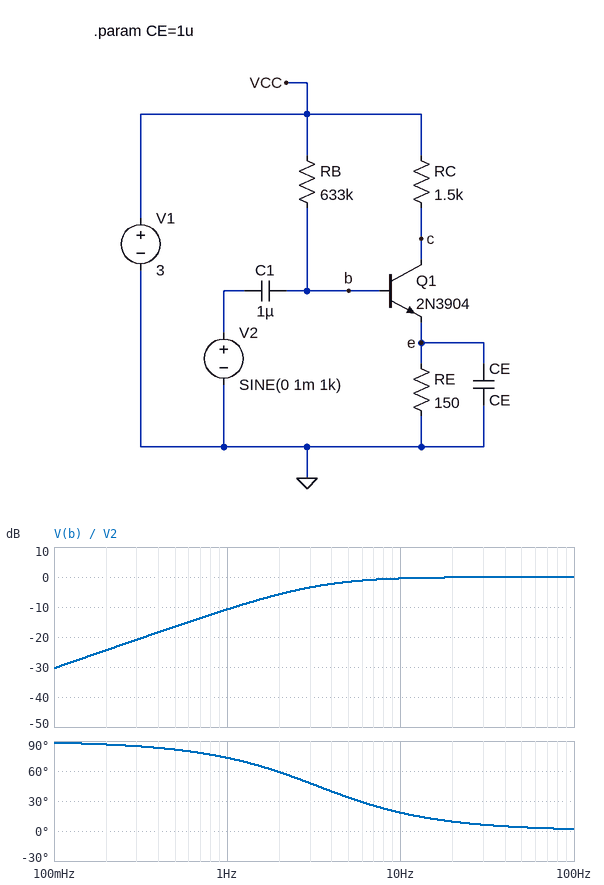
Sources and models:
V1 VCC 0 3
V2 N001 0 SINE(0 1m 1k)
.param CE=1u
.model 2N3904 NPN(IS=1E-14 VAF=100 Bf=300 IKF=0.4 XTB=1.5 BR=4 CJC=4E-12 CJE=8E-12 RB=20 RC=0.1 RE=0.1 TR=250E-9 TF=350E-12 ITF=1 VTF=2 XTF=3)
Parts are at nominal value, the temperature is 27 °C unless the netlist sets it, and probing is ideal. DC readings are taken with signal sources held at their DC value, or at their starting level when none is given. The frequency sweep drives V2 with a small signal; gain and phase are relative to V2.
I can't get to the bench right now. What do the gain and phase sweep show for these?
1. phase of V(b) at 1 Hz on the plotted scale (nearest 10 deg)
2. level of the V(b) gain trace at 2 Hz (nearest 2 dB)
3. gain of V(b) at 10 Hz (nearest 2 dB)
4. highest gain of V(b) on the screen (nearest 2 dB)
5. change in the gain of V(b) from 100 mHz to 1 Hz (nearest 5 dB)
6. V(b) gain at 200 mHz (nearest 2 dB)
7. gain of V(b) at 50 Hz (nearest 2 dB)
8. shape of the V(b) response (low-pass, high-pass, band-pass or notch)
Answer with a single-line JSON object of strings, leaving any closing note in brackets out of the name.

{"phase of V(b) at 1 Hz on the plotted scale": "70 deg", "level of the V(b) gain trace at 2 Hz": "-6 dB", "gain of V(b) at 10 Hz": "0 dB", "highest gain of V(b) on the screen": "0 dB", "change in the gain of V(b) from 100 mHz to 1 Hz": "20 dB", "V(b) gain at 200 mHz": "-24 dB", "gain of V(b) at 50 Hz": "0 dB", "shape of the V(b) response": "high-pass"}
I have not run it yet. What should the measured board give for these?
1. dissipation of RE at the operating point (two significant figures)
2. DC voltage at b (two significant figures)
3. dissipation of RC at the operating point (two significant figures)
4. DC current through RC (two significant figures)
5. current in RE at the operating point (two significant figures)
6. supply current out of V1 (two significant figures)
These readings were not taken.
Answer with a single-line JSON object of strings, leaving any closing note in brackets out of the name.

{"dissipation of RE at the operating point": "160 µW", "DC voltage at b": "810 mV", "dissipation of RC at the operating point": "1.6 mW", "DC current through RC": "1.0 mA", "current in RE at the operating point": "1.0 mA", "supply current out of V1": "1.0 mA"}
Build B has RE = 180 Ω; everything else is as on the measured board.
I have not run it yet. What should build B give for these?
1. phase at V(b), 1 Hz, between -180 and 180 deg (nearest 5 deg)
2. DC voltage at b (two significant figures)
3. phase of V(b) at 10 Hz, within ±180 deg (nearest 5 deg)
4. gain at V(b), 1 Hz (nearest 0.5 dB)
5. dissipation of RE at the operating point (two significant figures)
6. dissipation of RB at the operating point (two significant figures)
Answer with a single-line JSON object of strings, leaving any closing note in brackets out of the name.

{"phase at V(b), 1 Hz, between -180 and 180 deg": "70 deg", "DC voltage at b": "840 mV", "phase of V(b) at 10 Hz, within ±180 deg": "15 deg", "gain at V(b), 1 Hz": "-9.5 dB", "dissipation of RE at the operating point": "190 µW", "dissipation of RB at the operating point": "7.4 µW"}
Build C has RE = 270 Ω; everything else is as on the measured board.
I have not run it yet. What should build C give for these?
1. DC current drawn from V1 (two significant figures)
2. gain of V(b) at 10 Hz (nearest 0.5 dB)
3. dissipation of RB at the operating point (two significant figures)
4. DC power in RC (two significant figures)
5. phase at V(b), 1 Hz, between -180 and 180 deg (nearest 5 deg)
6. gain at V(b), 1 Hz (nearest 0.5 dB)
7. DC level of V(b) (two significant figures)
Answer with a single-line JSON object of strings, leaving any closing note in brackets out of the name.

{"DC current drawn from V1": "990 µA", "gain of V(b) at 10 Hz": "0 dB", "dissipation of RB at the operating point": "6.8 µW", "DC power in RC": "1.5 mW", "phase at V(b), 1 Hz, between -180 and 180 deg": "65 deg", "gain at V(b), 1 Hz": "-7.0 dB", "DC level of V(b)": "920 mV"}
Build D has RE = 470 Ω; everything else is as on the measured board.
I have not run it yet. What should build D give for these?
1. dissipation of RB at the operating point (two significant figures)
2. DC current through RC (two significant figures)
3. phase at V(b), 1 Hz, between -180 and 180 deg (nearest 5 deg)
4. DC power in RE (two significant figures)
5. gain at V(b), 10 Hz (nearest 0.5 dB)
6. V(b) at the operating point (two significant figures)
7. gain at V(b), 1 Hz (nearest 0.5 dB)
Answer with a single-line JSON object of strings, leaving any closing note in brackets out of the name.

{"dissipation of RB at the operating point": "5.8 µW", "DC current through RC": "910 µA", "phase at V(b), 1 Hz, between -180 and 180 deg": "55 deg", "DC power in RE": "390 µW", "gain at V(b), 10 Hz": "0 dB", "V(b) at the operating point": "1.1 V", "gain at V(b), 1 Hz": "-4.5 dB"}
